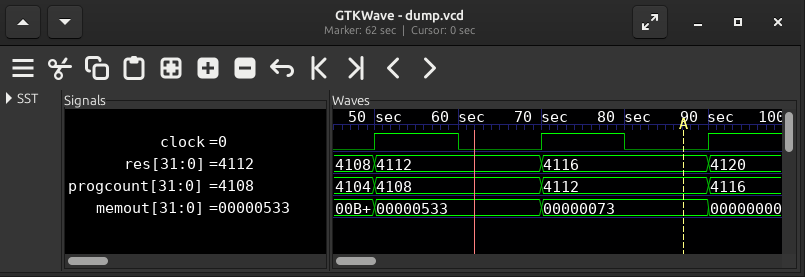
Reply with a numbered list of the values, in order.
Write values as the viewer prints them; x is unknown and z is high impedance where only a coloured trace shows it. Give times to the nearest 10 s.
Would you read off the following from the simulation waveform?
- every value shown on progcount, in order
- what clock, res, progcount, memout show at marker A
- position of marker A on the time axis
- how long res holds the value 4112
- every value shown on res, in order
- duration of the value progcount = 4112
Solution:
1. 4104, 4108, 4112, 4116
2. clock=0, res=4116, progcount=4112, memout=00000073
3. 90 s
4. 20 s
5. 4108, 4112, 4116, 4120
6. 20 s
